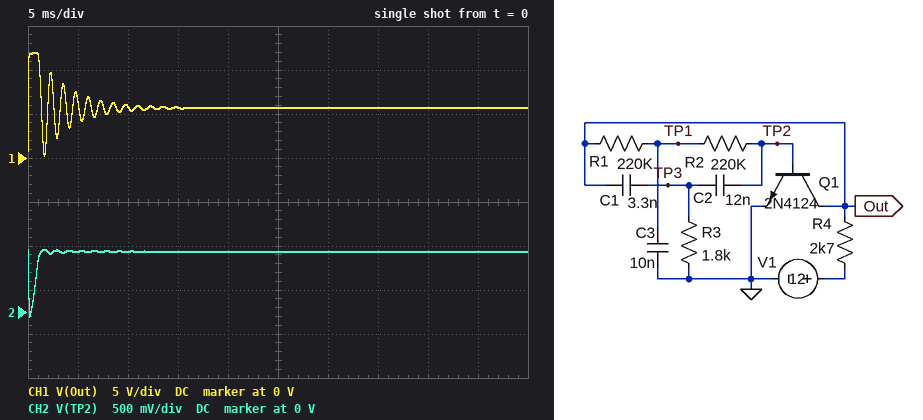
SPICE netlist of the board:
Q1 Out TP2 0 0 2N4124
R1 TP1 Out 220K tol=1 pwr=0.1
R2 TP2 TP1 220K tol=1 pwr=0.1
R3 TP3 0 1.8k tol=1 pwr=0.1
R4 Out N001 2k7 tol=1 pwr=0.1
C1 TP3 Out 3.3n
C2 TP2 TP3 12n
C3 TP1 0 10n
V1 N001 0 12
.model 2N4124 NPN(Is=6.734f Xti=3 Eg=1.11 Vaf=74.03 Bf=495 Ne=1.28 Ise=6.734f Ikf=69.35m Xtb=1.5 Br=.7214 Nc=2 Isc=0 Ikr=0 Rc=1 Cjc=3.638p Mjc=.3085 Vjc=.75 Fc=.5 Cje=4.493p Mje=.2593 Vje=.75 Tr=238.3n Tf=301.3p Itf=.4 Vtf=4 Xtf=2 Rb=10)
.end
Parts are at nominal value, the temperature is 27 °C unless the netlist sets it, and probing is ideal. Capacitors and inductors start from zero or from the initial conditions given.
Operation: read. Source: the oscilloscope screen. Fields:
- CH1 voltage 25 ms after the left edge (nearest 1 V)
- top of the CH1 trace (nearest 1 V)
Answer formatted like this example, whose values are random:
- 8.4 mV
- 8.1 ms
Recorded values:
- 6 V
- 12 V
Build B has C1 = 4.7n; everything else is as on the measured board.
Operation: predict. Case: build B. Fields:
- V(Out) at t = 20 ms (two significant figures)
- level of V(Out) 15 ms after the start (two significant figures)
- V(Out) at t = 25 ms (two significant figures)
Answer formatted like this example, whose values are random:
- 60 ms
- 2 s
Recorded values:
- 6.0 V
- 5.0 V
- 5.5 V
